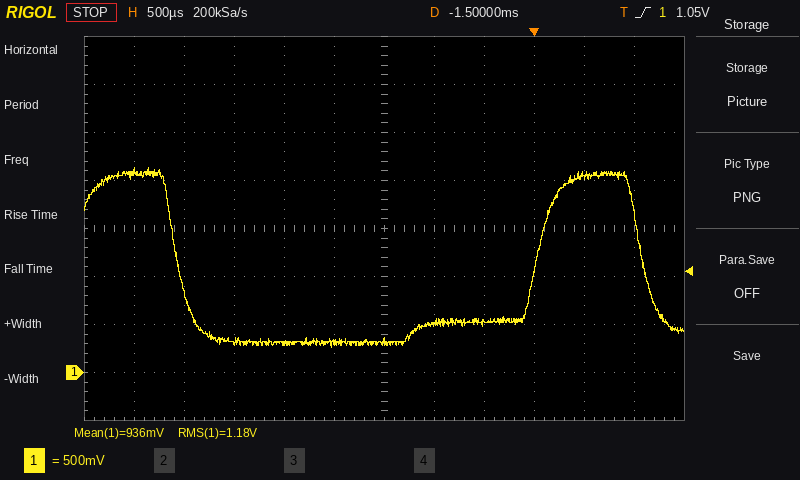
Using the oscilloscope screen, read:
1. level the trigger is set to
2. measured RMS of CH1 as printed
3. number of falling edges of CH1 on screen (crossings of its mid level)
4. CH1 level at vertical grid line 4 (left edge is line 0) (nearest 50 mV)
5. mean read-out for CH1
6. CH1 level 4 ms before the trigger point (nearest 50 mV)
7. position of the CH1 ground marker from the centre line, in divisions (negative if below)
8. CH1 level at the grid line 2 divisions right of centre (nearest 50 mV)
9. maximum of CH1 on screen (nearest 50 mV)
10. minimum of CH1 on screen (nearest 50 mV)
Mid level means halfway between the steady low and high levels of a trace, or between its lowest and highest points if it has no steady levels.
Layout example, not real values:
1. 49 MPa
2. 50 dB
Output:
1. 1.05 V
2. 1.18 V
3. 2
4. 300 mV
5. 936 mV
6. 2.10 V
7. -3.0 div
8. 500 mV
9. 2.15 V
10. 250 mV
